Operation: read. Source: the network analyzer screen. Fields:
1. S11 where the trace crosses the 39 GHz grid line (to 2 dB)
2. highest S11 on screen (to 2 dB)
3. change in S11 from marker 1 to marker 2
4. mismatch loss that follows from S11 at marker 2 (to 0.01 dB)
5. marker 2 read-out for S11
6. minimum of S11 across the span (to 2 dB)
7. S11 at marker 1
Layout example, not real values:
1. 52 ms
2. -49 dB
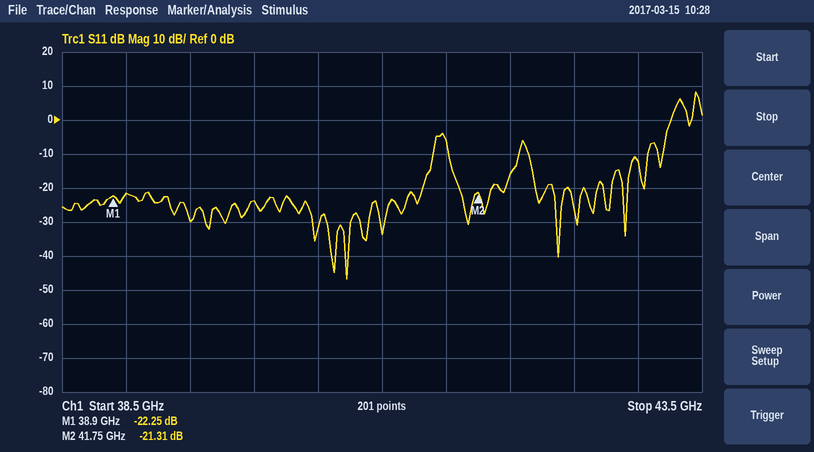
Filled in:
1. -22 dB
2. 8 dB
3. 0.94 dB
4. 0.03 dB
5. -21.31 dB
6. -46 dB
7. -22.25 dB
